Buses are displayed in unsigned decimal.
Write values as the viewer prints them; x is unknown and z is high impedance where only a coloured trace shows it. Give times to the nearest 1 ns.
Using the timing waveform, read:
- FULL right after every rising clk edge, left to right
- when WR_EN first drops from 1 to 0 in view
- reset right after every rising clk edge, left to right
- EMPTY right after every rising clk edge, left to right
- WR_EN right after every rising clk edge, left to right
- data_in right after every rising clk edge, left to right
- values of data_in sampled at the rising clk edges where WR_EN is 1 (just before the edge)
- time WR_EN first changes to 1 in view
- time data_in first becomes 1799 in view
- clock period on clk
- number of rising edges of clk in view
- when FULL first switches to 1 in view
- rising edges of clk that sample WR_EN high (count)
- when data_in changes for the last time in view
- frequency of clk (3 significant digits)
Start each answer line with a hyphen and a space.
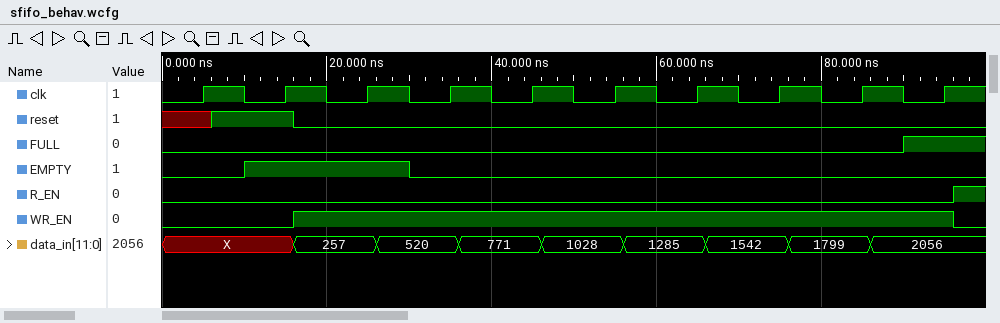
- 0 0 0 0 0 0 0 0 0 1
- 96 ns
- x 1 0 0 0 0 0 0 0 0
- 0 1 1 0 0 0 0 0 0 0
- 0 0 1 1 1 1 1 1 1 1
- X, X, 257, 520, 771, 1028, 1285, 1542, 1799, 2056
- 257, 520, 771, 1028, 1285, 1542, 1799, 2056
- 16 ns
- 76 ns
- 10 ns
- 10
- 90 ns
- 8
- 86 ns
- 100 MHz
